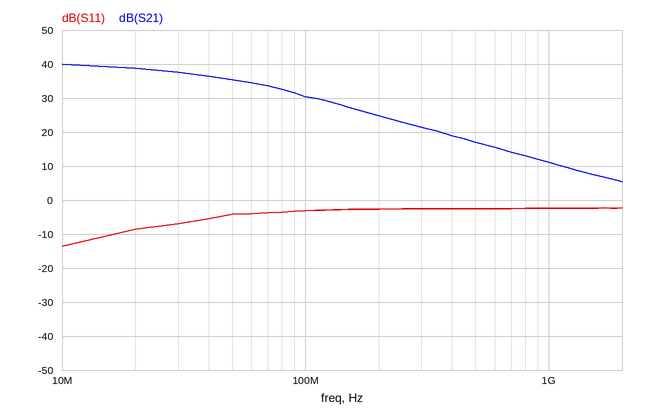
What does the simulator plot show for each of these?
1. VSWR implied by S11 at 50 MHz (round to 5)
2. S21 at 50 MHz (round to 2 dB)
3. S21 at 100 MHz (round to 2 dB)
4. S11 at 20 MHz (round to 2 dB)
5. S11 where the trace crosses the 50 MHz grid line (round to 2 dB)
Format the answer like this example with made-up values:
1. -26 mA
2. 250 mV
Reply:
1. 5
2. 36 dB
3. 30 dB
4. -8 dB
5. -4 dB
